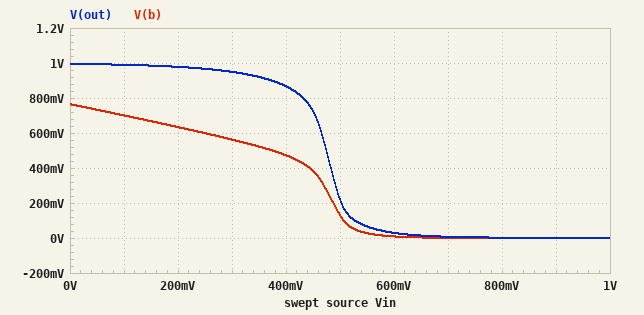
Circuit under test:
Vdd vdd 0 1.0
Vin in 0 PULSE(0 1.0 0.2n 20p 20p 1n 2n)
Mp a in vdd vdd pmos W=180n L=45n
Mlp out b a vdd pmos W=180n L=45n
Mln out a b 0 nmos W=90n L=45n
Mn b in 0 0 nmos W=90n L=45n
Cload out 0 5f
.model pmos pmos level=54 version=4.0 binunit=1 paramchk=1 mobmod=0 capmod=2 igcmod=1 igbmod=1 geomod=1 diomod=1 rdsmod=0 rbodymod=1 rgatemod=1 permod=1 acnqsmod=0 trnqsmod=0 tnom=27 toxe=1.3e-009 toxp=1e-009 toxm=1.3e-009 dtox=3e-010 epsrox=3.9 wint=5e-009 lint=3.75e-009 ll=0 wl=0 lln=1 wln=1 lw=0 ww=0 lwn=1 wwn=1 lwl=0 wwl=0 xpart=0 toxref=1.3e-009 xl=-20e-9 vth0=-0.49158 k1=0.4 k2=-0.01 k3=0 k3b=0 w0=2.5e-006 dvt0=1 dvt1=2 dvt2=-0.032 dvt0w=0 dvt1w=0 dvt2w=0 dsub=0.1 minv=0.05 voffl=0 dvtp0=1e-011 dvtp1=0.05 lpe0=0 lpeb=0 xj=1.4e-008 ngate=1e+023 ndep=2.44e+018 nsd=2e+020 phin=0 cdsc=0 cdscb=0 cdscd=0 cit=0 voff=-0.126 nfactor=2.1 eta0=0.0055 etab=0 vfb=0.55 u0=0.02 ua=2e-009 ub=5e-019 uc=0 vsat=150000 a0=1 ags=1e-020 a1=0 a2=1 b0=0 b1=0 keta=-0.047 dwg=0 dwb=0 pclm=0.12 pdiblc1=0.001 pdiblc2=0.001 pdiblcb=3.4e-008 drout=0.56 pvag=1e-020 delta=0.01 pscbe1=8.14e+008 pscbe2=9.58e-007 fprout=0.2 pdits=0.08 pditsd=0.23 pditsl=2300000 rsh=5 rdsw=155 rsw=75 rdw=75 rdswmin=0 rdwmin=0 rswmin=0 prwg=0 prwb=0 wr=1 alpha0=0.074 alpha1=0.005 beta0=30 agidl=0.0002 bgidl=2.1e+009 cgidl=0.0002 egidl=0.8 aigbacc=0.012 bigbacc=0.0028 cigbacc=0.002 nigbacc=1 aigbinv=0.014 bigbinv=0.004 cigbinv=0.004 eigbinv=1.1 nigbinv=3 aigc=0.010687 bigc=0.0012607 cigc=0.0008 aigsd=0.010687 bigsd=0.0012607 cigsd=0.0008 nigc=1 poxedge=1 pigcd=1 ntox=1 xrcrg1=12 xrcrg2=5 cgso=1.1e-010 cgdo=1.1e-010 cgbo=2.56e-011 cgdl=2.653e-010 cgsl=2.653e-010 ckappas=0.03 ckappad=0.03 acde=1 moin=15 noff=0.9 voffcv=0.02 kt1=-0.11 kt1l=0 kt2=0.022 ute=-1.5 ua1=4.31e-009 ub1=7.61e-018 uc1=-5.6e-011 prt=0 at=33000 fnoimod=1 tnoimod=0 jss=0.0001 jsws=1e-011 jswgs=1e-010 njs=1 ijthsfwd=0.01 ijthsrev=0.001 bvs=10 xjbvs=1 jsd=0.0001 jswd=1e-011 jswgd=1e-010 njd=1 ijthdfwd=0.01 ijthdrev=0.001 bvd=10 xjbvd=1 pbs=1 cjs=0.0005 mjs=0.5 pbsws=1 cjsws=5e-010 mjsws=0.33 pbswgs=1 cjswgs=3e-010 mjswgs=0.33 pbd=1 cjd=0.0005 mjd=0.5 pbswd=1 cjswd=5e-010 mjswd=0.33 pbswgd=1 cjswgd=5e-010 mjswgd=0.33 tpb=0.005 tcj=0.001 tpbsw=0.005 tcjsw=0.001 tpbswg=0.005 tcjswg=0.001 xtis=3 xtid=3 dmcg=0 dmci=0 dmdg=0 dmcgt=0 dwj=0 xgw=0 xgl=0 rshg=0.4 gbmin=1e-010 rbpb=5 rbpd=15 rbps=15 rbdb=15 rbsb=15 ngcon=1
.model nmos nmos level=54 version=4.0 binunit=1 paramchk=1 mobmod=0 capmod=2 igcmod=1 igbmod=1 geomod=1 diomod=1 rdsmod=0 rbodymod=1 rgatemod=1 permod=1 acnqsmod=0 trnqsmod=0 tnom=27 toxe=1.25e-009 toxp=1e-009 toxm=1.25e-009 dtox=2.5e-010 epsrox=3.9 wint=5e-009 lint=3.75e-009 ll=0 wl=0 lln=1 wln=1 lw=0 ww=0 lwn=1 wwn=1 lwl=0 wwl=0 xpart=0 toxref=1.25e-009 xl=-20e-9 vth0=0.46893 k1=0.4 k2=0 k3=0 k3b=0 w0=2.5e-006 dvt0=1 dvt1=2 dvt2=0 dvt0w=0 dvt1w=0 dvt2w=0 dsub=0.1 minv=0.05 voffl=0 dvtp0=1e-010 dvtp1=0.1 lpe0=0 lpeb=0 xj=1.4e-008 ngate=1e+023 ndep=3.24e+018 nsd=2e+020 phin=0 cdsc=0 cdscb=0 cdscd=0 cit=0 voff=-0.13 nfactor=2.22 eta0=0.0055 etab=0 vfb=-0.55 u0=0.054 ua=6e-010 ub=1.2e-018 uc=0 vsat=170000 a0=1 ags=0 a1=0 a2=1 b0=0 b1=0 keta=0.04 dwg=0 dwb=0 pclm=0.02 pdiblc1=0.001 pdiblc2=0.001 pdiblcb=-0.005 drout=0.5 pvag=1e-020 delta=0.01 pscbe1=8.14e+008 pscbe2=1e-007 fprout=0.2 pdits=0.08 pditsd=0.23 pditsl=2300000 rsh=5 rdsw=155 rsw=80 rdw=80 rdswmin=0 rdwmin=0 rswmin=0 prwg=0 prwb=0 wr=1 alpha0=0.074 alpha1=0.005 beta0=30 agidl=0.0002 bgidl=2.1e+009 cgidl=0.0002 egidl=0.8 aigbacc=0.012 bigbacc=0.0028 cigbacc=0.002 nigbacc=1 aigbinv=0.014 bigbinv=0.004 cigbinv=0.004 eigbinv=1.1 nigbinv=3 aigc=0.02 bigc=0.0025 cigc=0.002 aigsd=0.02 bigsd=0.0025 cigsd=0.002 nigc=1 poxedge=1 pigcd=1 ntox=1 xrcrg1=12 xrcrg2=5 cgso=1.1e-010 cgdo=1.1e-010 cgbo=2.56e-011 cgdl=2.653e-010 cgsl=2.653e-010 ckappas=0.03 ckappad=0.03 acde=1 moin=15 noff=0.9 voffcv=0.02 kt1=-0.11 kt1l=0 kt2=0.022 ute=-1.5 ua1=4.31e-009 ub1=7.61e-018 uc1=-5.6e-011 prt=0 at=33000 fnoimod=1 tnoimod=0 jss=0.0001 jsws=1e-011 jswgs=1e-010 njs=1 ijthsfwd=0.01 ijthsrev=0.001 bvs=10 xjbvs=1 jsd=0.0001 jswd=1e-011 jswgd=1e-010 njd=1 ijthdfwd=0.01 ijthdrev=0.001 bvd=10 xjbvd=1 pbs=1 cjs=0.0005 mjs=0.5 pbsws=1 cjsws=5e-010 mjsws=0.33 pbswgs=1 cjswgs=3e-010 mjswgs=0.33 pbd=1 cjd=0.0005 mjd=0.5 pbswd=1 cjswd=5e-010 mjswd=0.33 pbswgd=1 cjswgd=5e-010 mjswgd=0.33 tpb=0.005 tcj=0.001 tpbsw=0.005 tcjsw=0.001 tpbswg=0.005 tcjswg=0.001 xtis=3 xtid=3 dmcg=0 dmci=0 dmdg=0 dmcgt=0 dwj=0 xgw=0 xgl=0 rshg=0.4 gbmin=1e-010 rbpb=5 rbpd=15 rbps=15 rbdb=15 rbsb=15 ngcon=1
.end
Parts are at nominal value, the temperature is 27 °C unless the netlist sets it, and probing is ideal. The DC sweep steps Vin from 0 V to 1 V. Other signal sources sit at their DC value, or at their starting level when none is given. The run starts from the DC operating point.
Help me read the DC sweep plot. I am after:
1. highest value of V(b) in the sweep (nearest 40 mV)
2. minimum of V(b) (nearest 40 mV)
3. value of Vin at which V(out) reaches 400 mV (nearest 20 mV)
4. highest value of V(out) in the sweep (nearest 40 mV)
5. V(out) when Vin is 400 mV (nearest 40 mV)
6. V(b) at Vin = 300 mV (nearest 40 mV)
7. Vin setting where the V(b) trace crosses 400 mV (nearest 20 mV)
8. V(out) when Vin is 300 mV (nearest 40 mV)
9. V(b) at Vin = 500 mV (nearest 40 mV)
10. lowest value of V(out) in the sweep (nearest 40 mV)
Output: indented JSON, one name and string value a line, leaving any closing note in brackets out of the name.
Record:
{
  "highest value of V(b) in the sweep": "760 mV",
  "minimum of V(b)": "0 V",
  "value of Vin at which V(out) reaches 400 mV": "480 mV",
  "highest value of V(out) in the sweep": "1.00 V",
  "V(out) when Vin is 400 mV": "880 mV",
  "V(b) at Vin = 300 mV": "560 mV",
  "Vin setting where the V(b) trace crosses 400 mV": "440 mV",
  "V(out) when Vin is 300 mV": "960 mV",
  "V(b) at Vin = 500 mV": "120 mV",
  "lowest value of V(out) in the sweep": "0 V"
}
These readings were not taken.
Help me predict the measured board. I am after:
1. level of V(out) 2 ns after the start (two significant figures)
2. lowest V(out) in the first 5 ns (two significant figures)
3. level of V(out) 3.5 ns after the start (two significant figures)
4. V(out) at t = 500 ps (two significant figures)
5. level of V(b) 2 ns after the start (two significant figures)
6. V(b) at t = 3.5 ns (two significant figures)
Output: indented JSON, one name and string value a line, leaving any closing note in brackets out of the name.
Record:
{
  "level of V(out) 2 ns after the start": "680 mV",
  "lowest V(out) in the first 5 ns": "120 mV",
  "level of V(out) 3.5 ns after the start": "620 mV",
  "V(out) at t = 500 ps": "280 mV",
  "level of V(b) 2 ns after the start": "640 mV",
  "V(b) at t = 3.5 ns": "590 mV"
}
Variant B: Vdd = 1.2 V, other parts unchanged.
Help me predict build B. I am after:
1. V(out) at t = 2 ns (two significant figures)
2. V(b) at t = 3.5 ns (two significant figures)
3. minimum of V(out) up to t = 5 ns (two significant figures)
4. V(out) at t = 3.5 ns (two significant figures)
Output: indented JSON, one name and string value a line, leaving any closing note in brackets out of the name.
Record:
{
  "V(out) at t = 2 ns": "910 mV",
  "V(b) at t = 3.5 ns": "780 mV",
  "minimum of V(out) up to t = 5 ns": "16 mV",
  "V(out) at t = 3.5 ns": "830 mV"
}
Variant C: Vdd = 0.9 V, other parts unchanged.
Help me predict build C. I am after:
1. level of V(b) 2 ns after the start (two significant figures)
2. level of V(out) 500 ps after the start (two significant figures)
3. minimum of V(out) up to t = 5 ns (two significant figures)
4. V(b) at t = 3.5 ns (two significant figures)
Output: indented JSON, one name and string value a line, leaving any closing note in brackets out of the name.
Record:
{
  "level of V(b) 2 ns after the start": "550 mV",
  "level of V(out) 500 ps after the start": "300 mV",
  "minimum of V(out) up to t = 5 ns": "150 mV",
  "V(b) at t = 3.5 ns": "490 mV"
}
